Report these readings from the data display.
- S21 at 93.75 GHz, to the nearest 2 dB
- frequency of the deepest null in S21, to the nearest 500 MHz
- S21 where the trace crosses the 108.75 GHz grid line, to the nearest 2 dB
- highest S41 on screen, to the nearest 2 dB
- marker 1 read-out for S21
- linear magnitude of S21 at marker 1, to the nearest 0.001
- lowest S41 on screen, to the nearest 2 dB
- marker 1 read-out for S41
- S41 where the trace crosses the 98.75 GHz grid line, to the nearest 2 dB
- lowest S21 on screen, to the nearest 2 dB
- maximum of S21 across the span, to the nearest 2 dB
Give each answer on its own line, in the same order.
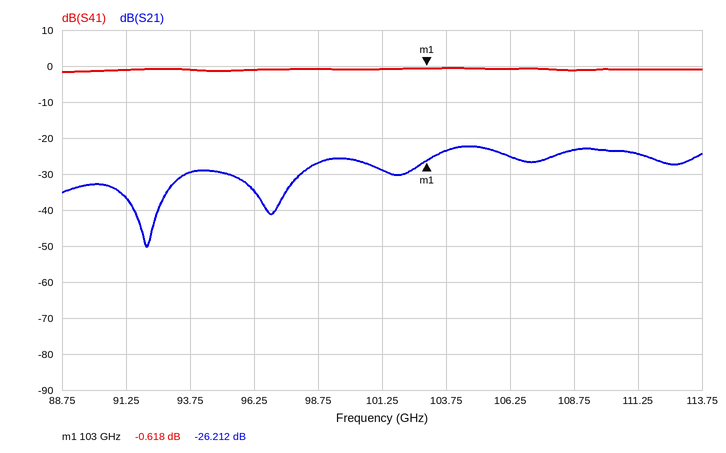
-30 dB
92.0 GHz
-24 dB
0 dB
-26.212 dB
0.049
-2 dB
-0.618 dB
0 dB
-50 dB
-22 dB
